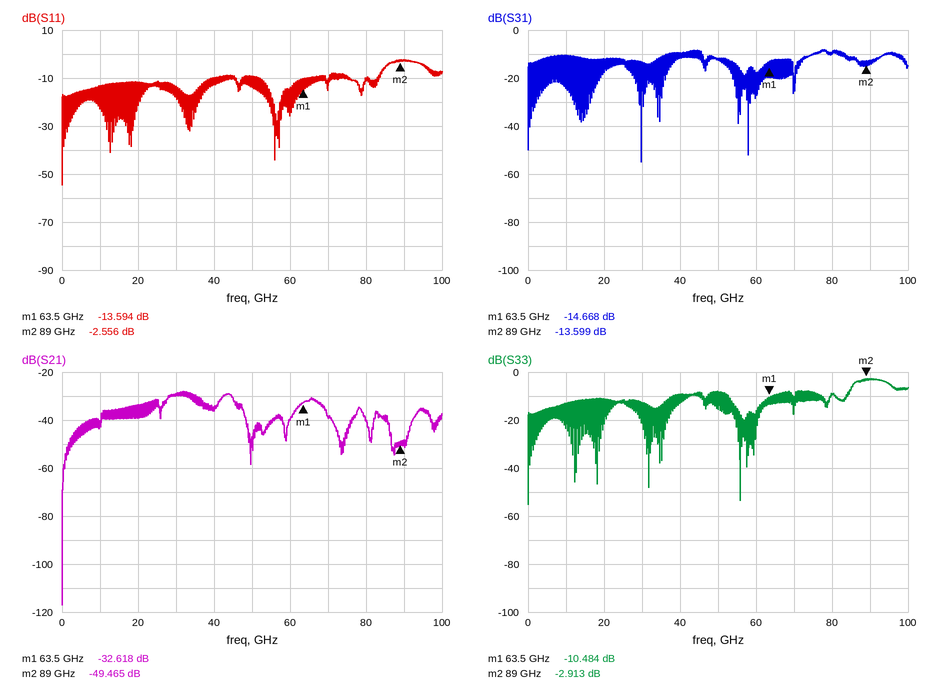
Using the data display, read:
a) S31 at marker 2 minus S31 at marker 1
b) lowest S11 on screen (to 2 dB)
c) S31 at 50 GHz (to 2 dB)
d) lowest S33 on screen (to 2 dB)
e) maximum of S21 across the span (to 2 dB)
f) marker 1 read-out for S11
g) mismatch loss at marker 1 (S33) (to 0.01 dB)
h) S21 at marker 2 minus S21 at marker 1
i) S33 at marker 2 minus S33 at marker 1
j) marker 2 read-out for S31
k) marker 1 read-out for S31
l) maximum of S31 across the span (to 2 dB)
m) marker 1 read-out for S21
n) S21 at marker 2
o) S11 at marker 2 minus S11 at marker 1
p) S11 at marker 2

1.069 dB
-54 dB
-12 dB
-56 dB
-28 dB
-13.594 dB
0.41 dB
-16.847 dB
7.571 dB
-13.599 dB
-14.668 dB
-8 dB
-32.618 dB
-49.465 dB
11.038 dB
-2.556 dB
